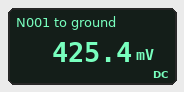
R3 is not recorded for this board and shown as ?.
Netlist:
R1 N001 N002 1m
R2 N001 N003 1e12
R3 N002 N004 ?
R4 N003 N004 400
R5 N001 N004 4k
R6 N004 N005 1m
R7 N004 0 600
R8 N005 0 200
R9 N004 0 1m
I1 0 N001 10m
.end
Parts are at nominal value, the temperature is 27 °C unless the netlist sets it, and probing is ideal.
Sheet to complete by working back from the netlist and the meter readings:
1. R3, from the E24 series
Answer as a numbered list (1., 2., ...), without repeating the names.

1. 43 Ω
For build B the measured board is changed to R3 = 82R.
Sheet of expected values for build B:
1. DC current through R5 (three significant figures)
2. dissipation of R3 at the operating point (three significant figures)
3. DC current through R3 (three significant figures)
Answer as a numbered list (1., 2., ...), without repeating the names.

1. 201 µA
2. 7.87 mW
3. 9.80 mA
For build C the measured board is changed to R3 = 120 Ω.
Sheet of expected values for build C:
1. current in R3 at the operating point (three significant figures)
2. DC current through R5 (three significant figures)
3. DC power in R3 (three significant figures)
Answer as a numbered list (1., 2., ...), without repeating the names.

1. 9.71 mA
2. 291 µA
3. 11.3 mW
